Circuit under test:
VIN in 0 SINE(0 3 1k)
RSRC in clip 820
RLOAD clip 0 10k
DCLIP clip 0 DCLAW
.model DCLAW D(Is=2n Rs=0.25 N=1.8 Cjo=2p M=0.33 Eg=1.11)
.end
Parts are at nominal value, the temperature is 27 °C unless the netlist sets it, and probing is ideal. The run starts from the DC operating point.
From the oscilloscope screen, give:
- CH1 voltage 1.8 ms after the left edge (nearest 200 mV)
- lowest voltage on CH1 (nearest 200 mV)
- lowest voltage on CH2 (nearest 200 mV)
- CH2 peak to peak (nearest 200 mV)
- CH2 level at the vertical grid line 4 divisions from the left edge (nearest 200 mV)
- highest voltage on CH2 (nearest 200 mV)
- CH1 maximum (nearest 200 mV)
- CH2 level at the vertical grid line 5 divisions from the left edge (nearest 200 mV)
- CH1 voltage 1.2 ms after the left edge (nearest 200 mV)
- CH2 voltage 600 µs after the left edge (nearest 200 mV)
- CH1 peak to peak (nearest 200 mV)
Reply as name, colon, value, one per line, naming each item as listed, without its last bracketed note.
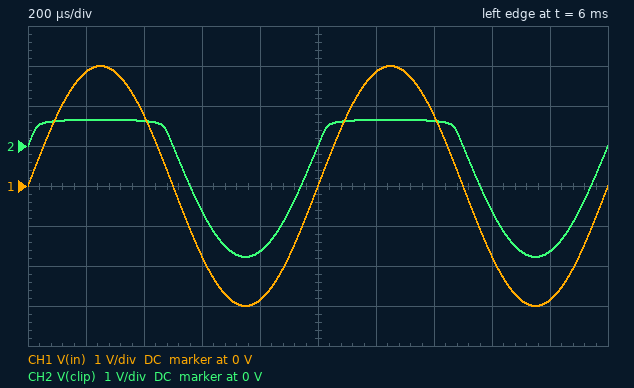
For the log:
CH1 voltage 1.8 ms after the left edge: -2.8 V
lowest voltage on CH1: -3.0 V
lowest voltage on CH2: -2.8 V
CH2 peak to peak: 3.4 V
CH2 level at the vertical grid line 4 divisions from the left edge: -2.6 V
highest voltage on CH2: 600 mV
CH1 maximum: 3.0 V
CH2 level at the vertical grid line 5 divisions from the left edge: 0 V
CH1 voltage 1.2 ms after the left edge: 2.8 V
CH2 voltage 600 µs after the left edge: -1.6 V
CH1 peak to peak: 6.0 V
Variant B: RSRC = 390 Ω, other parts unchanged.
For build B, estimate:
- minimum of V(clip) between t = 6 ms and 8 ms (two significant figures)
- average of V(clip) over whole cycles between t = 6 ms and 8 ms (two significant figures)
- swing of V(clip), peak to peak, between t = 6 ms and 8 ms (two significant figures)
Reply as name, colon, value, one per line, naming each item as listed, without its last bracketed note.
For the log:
minimum of V(clip) between t = 6 ms and 8 ms: -2.9 V
average of V(clip) over whole cycles between t = 6 ms and 8 ms: -610 mV
swing of V(clip), peak to peak, between t = 6 ms and 8 ms: 3.6 V
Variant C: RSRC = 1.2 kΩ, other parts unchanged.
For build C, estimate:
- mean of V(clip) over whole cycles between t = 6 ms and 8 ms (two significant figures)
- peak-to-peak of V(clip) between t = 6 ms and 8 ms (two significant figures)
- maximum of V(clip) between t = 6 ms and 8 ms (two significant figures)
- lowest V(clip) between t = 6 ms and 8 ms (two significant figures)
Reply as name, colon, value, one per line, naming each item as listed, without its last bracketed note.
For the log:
mean of V(clip) over whole cycles between t = 6 ms and 8 ms: -570 mV
peak-to-peak of V(clip) between t = 6 ms and 8 ms: 3.3 V
maximum of V(clip) between t = 6 ms and 8 ms: 640 mV
lowest V(clip) between t = 6 ms and 8 ms: -2.7 V
